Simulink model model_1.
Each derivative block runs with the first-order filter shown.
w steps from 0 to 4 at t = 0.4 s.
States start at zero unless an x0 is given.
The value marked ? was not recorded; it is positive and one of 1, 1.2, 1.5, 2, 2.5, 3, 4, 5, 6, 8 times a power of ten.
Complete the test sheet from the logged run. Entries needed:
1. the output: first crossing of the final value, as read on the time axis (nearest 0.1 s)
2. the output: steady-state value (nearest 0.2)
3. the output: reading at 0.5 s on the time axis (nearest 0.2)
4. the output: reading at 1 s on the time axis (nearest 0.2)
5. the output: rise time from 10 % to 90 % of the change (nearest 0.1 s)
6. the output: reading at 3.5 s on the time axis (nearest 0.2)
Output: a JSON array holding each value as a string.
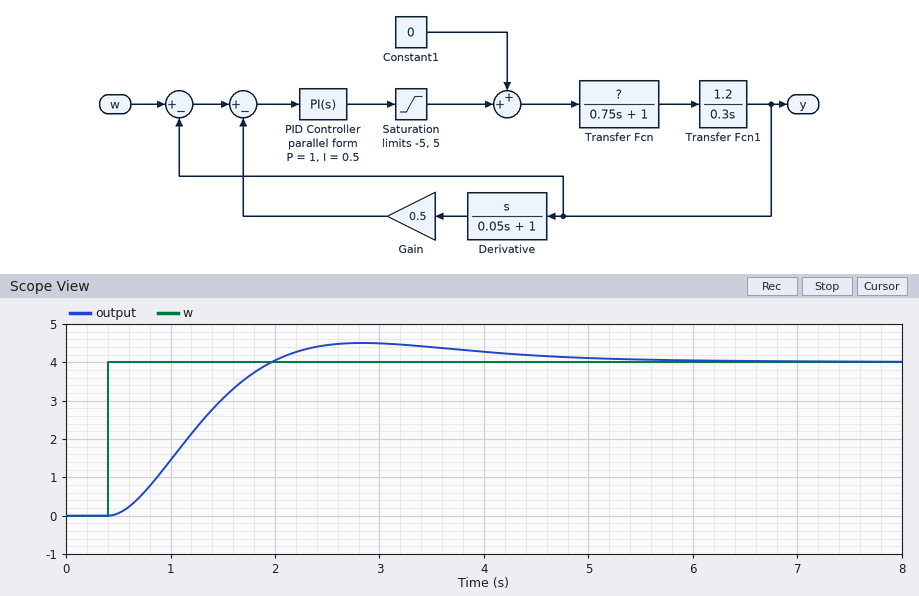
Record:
["2.0 s", "4.0", "0.0", "1.4", "1.1 s", "4.4"]
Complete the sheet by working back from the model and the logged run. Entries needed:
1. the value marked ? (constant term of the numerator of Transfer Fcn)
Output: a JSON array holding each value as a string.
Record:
["0.6"]
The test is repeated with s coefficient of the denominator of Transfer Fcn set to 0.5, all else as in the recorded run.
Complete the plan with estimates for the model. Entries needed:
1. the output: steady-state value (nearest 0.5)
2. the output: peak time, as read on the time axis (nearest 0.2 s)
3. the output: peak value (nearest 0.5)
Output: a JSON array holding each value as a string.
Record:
["4.0", "3.2 s", "4.5"]
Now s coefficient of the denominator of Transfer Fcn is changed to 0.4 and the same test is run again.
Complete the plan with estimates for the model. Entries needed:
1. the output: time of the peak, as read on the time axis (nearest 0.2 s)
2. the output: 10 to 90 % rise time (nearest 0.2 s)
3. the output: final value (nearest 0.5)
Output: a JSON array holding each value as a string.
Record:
["3.4 s", "1.2 s", "4.0"]
